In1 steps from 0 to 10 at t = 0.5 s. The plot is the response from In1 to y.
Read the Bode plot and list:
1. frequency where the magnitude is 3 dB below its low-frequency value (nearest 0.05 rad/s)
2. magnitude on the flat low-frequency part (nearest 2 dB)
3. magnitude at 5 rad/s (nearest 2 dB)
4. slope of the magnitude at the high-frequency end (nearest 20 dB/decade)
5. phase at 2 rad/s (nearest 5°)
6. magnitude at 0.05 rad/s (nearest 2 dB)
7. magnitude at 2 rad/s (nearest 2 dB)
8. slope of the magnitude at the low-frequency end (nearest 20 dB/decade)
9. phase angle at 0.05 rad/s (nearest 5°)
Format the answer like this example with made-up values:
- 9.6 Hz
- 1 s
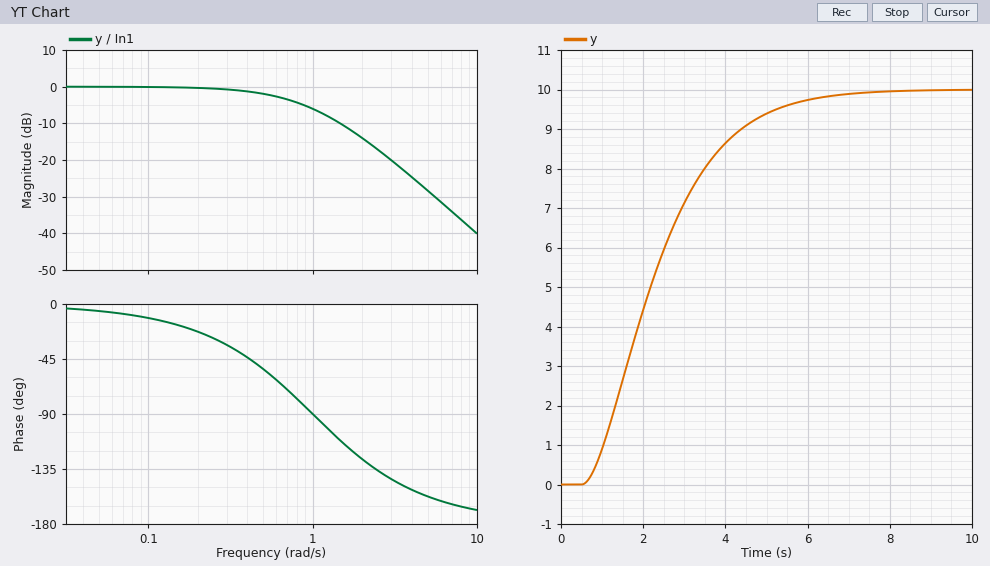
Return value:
- 0.65 rad/s
- 0 dB
- -28 dB
- -40 dB/decade
- -125°
- 0 dB
- -14 dB
- 0 dB/decade
- -5°
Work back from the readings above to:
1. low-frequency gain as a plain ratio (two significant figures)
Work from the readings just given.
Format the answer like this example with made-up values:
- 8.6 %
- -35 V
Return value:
- 1.0
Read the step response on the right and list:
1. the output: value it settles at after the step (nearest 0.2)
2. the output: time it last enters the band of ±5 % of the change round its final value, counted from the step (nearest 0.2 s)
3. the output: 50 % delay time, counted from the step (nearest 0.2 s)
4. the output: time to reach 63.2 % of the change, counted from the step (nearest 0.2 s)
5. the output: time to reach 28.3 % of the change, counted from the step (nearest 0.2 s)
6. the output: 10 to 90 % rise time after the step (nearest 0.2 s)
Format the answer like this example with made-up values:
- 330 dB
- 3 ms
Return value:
- 10.0
- 4.8 s
- 1.6 s
- 2.2 s
- 1.0 s
- 3.4 s
